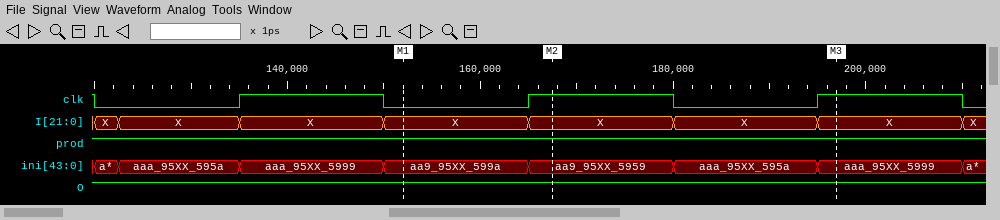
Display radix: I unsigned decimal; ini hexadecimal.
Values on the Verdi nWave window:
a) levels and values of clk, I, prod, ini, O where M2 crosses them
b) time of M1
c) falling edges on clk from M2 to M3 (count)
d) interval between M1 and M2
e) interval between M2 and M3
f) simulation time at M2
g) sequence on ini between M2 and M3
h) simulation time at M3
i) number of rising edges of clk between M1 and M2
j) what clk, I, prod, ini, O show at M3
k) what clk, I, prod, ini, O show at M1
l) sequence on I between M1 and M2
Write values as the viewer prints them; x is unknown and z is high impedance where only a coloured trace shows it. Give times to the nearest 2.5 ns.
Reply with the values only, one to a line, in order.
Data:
clk=1, I=X, prod=1, ini=aa9_95XX_5959, O=1
152.5 ns
1
15 ns
30 ns
167.5 ns
aa9_95XX_5959, aaa_95XX_595a, aaa_95XX_5999
197.5 ns
1
clk=1, I=X, prod=1, ini=aaa_95XX_5999, O=1
clk=0, I=X, prod=1, ini=aa9_95XX_599a, O=1
X, X
